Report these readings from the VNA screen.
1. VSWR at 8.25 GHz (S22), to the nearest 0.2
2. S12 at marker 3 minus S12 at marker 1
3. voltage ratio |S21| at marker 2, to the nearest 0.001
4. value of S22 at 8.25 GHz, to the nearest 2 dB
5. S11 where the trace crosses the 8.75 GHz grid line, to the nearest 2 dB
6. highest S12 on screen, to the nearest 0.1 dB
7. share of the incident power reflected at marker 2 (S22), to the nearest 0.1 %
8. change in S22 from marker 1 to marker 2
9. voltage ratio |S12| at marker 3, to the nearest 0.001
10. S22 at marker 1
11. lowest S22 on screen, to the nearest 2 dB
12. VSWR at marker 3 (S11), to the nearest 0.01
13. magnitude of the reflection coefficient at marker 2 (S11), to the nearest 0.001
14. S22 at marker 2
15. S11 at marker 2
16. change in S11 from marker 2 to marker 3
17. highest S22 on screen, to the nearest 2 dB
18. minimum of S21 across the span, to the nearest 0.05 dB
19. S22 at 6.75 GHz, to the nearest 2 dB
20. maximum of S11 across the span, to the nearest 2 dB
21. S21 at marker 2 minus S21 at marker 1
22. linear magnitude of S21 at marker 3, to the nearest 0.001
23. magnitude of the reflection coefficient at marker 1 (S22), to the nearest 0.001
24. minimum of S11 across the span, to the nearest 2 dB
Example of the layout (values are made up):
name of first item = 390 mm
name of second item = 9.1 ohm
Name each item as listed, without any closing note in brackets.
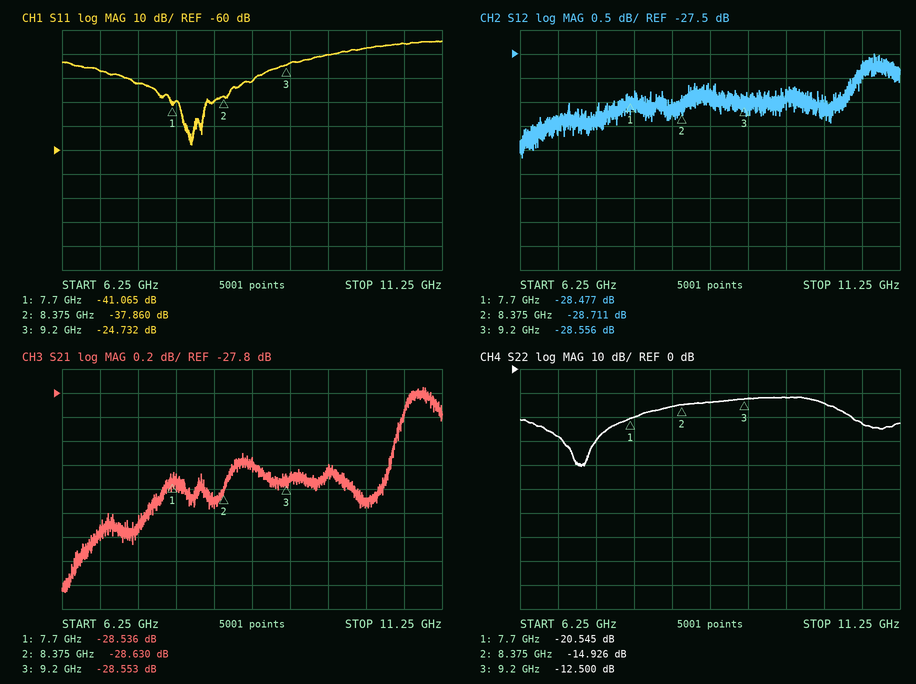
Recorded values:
VSWR at 8.25 GHz (S22), to the nearest 0.2 = 1.4
S12 at marker 3 minus S12 at marker 1 = -0.079 dB
voltage ratio |S21| at marker 2, to the nearest 0.001 = 0.037
value of S22 at 8.25 GHz, to the nearest 2 dB = -16 dB
S11 where the trace crosses the 8.75 GHz grid line, to the nearest 2 dB = -32 dB
highest S12 on screen, to the nearest 0.1 dB = -27.5 dB
share of the incident power reflected at marker 2 (S22), to the nearest 0.1 % = 3.2 %
change in S22 from marker 1 to marker 2 = 5.619 dB
voltage ratio |S12| at marker 3, to the nearest 0.001 = 0.037
S22 at marker 1 = -20.545 dB
lowest S22 on screen, to the nearest 2 dB = -40 dB
VSWR at marker 3 (S11), to the nearest 0.01 = 1.12
magnitude of the reflection coefficient at marker 2 (S11), to the nearest 0.001 = 0.013
S22 at marker 2 = -14.926 dB
S11 at marker 2 = -37.860 dB
change in S11 from marker 2 to marker 3 = 13.128 dB
highest S22 on screen, to the nearest 2 dB = -12 dB
minimum of S21 across the span, to the nearest 0.05 dB = -29.45 dB
S22 at 6.75 GHz, to the nearest 2 dB = -28 dB
maximum of S11 across the span, to the nearest 2 dB = -14 dB
S21 at marker 2 minus S21 at marker 1 = -0.094 dB
linear magnitude of S21 at marker 3, to the nearest 0.001 = 0.037
magnitude of the reflection coefficient at marker 1 (S22), to the nearest 0.001 = 0.094
minimum of S11 across the span, to the nearest 2 dB = -58 dB
